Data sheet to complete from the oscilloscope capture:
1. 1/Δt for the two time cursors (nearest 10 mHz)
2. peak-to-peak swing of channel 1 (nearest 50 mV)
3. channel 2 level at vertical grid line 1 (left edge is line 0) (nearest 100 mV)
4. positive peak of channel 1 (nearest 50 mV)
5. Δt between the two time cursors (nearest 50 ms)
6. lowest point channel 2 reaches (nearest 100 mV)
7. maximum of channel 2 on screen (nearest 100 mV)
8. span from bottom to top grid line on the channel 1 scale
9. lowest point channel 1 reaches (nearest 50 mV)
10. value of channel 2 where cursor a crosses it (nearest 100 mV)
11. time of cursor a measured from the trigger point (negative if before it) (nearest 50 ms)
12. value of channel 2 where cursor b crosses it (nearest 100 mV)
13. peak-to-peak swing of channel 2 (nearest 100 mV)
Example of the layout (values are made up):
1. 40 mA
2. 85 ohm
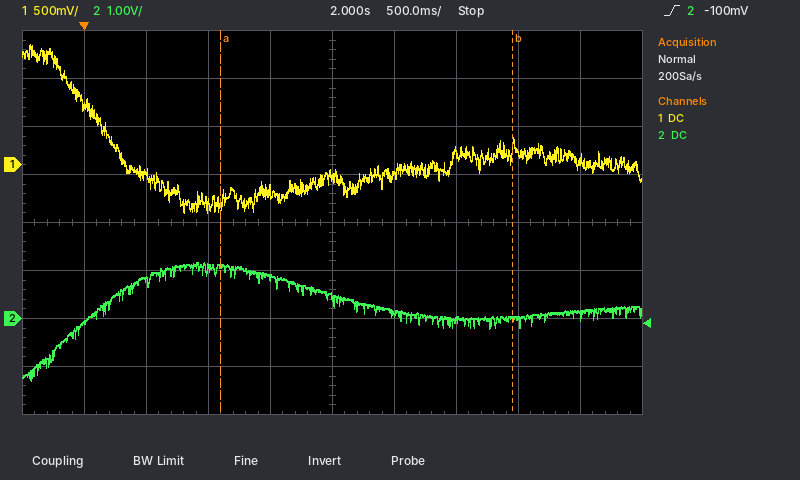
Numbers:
1. 430 mHz
2. 1.75 V
3. -100 mV
4. 1.25 V
5. 2.35 s
6. -1.3 V
7. 1.2 V
8. 4 V
9. -500 mV
10. 1.1 V
11. +1.10 s
12. 0.0 V
13. 2.5 V
